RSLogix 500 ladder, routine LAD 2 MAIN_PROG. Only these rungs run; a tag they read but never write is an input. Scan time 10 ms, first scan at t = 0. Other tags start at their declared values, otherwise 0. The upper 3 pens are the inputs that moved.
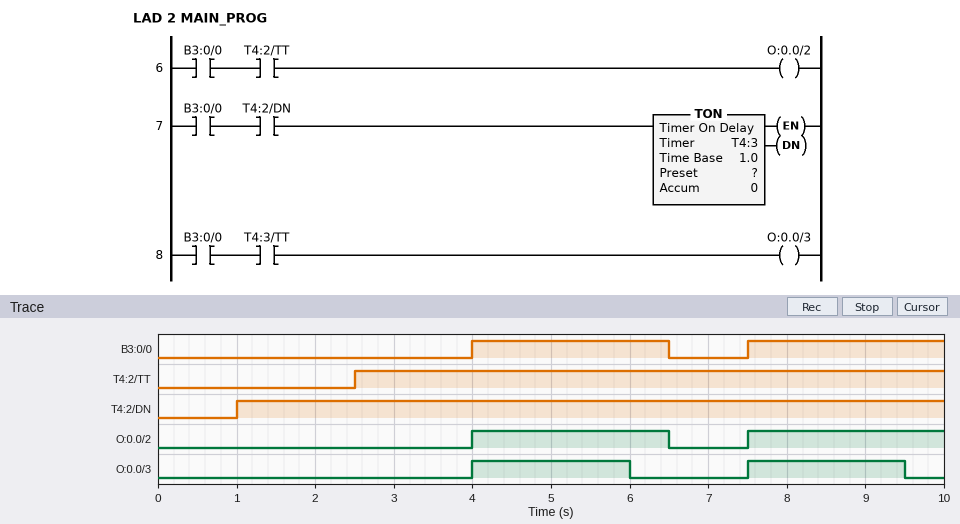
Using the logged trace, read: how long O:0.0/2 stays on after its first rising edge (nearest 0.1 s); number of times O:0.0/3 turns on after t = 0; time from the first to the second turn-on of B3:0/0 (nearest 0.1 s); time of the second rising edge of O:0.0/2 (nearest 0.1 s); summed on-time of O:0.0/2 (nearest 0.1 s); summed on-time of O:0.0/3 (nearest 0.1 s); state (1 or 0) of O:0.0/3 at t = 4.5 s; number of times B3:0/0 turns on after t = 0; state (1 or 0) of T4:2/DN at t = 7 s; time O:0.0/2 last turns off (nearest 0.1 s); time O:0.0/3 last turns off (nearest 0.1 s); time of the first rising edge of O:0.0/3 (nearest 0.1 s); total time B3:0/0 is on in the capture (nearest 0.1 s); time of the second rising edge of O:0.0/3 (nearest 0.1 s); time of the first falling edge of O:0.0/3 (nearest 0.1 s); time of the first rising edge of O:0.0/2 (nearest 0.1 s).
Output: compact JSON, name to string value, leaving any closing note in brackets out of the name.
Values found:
{"how long O:0.0/2 stays on after its first rising edge": "2.5 s", "number of times O:0.0/3 turns on after t = 0": "2", "time from the first to the second turn-on of B3:0/0": "3.5 s", "time of the second rising edge of O:0.0/2": "7.5 s", "summed on-time of O:0.0/2": "5.0 s", "summed on-time of O:0.0/3": "4.0 s", "state (1 or 0) of O:0.0/3 at t = 4.5 s": "1", "number of times B3:0/0 turns on after t = 0": "2", "state (1 or 0) of T4:2/DN at t = 7 s": "1", "time O:0.0/2 last turns off": "6.5 s", "time O:0.0/3 last turns off": "9.5 s", "time of the first rising edge of O:0.0/3": "4.0 s", "total time B3:0/0 is on in the capture": "5.0 s", "time of the second rising edge of O:0.0/3": "7.5 s", "time of the first falling edge of O:0.0/3": "6.0 s", "time of the first rising edge of O:0.0/2": "4.0 s"}
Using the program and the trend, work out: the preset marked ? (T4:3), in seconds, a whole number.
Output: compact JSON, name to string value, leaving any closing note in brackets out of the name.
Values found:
{"the preset marked ? (T4:3), in seconds, a whole number": "2 s"}
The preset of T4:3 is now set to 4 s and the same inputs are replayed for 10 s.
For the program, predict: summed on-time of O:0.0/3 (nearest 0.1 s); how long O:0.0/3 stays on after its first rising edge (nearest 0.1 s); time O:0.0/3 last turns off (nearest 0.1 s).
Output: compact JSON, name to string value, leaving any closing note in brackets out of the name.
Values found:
{"summed on-time of O:0.0/3": "5.0 s", "how long O:0.0/3 stays on after its first rising edge": "2.5 s", "time O:0.0/3 last turns off": "6.5 s"}
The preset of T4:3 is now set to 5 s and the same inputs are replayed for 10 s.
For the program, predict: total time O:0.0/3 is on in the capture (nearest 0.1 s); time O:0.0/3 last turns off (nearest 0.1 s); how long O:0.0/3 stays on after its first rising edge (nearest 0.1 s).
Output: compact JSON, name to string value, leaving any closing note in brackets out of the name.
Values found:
{"total time O:0.0/3 is on in the capture": "5.0 s", "time O:0.0/3 last turns off": "6.5 s", "how long O:0.0/3 stays on after its first rising edge": "2.5 s"}
